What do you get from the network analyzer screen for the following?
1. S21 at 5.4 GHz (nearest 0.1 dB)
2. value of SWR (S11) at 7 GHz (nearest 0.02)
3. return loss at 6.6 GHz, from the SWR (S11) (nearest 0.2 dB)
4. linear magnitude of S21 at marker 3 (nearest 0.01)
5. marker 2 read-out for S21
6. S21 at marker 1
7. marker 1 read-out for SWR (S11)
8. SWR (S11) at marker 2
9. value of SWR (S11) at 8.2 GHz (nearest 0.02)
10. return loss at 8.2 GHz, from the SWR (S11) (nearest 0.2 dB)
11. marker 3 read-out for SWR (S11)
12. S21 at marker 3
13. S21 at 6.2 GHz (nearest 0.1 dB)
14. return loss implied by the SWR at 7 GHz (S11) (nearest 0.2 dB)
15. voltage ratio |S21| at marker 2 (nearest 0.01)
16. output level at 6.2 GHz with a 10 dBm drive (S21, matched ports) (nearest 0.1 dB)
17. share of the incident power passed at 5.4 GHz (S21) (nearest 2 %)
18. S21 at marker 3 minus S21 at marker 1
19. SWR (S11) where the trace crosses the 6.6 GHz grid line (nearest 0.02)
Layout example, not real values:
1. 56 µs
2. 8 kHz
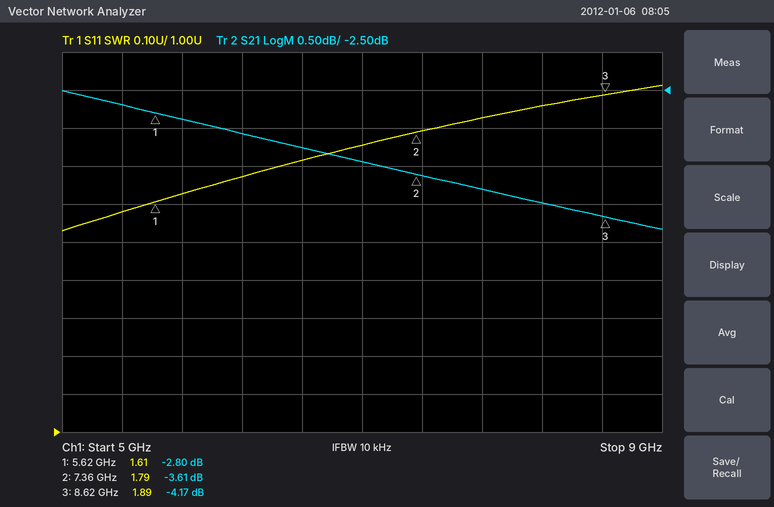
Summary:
1. -2.7 dB
2. 1.76
3. 11.6 dB
4. 0.62
5. -3.61 dB
6. -2.80 dB
7. 1.61
8. 1.79
9. 1.86
10. 10.4 dB
11. 1.89
12. -4.17 dB
13. -3.1 dB
14. 11.2 dB
15. 0.66
16. 6.9 dBm
17. 54 %
18. -1.37 dB
19. 1.72
